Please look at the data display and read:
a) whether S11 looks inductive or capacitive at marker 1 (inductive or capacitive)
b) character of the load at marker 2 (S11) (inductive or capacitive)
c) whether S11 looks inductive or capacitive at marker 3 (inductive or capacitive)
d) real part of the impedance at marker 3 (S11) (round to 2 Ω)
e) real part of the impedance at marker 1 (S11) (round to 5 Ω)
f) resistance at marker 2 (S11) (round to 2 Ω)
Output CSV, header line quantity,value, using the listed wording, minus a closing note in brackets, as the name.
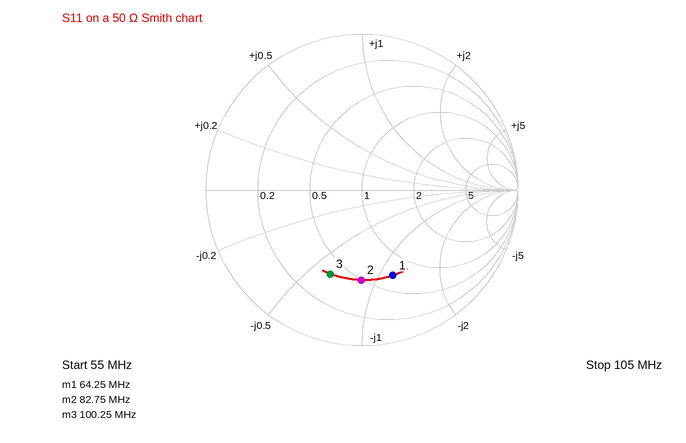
quantity,value
whether S11 looks inductive or capacitive at marker 1,capacitive
character of the load at marker 2 (S11),capacitive
whether S11 looks inductive or capacitive at marker 3,capacitive
real part of the impedance at marker 3 (S11),20 Ω
real part of the impedance at marker 1 (S11),35 Ω
resistance at marker 2 (S11),24 Ω
